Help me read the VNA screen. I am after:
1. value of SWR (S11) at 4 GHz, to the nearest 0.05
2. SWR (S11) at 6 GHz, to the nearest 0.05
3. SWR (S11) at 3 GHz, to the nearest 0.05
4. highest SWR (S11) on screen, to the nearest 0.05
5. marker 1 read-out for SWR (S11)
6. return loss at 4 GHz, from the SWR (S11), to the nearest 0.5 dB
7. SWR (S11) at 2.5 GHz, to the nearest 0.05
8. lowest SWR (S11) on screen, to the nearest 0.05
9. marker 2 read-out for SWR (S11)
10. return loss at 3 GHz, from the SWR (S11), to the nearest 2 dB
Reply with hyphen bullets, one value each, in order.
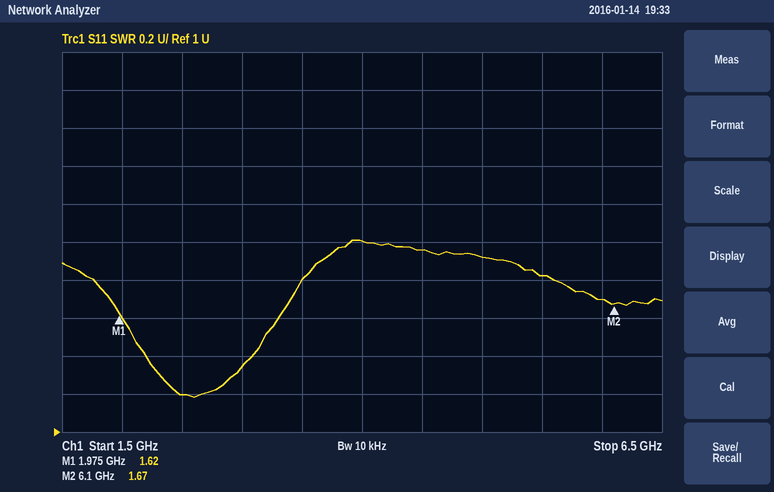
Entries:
- 2.00
- 1.70
- 1.35
- 2.00
- 1.62
- 9.5 dB
- 1.20
- 1.20
- 1.67
- 16 dB
